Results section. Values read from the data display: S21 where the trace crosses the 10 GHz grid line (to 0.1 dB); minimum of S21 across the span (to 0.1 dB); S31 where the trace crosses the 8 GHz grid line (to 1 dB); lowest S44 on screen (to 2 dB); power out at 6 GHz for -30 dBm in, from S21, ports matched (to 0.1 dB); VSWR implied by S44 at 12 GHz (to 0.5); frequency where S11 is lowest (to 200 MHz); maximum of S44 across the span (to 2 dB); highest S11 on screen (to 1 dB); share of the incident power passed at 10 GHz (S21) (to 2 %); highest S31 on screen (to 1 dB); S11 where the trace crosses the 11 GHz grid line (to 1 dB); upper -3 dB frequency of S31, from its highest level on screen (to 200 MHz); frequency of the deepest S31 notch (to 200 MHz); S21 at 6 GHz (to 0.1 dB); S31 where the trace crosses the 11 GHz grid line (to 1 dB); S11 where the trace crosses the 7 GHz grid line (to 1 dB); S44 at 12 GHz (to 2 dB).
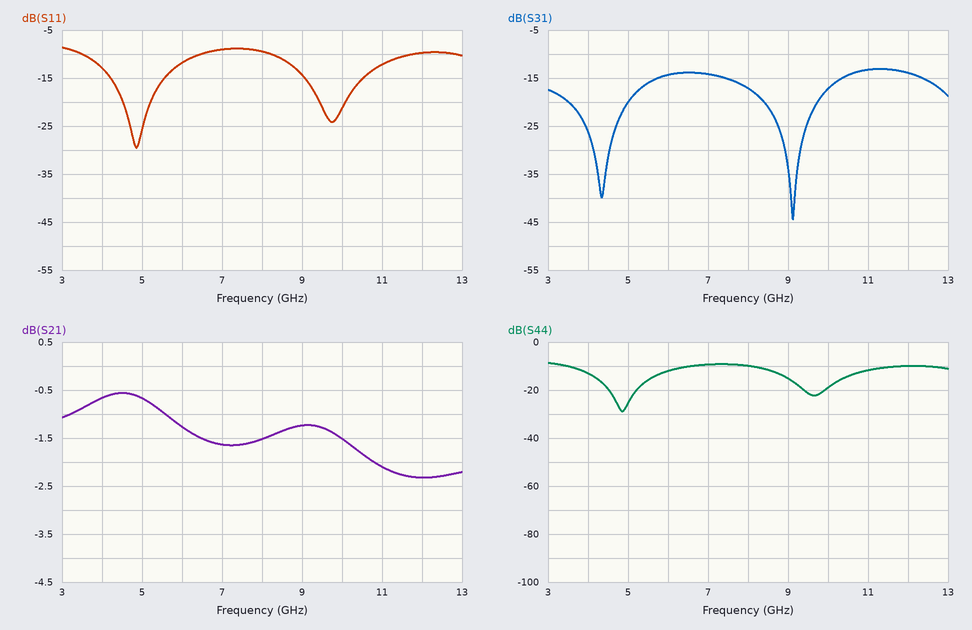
-1.5 dB
-2.3 dB
-17 dB
-28 dB
-31.3 dBm
2.0
4.8 GHz
-8 dB
-9 dB
70 %
-13 dB
-12 dB
12.6 GHz
9.2 GHz
-1.3 dB
-13 dB
-9 dB
-10 dB
